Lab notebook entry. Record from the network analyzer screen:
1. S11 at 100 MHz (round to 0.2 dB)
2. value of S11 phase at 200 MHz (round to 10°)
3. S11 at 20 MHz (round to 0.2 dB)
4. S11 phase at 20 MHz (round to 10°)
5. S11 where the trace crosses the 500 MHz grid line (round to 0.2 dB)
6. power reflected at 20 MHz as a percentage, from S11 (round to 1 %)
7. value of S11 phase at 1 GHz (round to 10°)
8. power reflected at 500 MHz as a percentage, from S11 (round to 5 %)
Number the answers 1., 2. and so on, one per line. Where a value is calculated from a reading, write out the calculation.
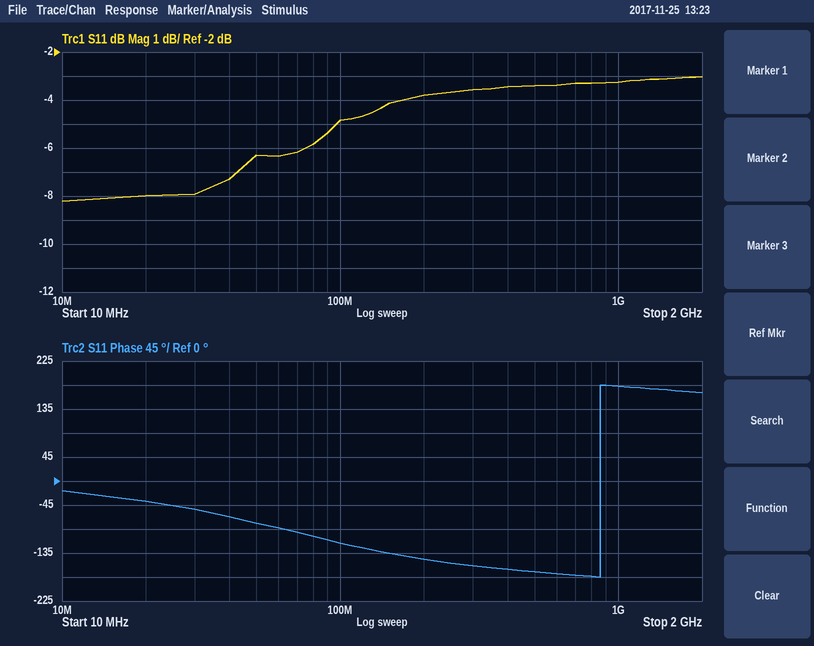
1. -4.8 dB
2. -150°
3. -8.0 dB
4. -40°
5. -3.4 dB
6. 10^(-8/10) ≈ 16 %
7. 180°
8. 10^(-3.4/10) ≈ 45.7 %, so 45 % to the nearest 5 %
